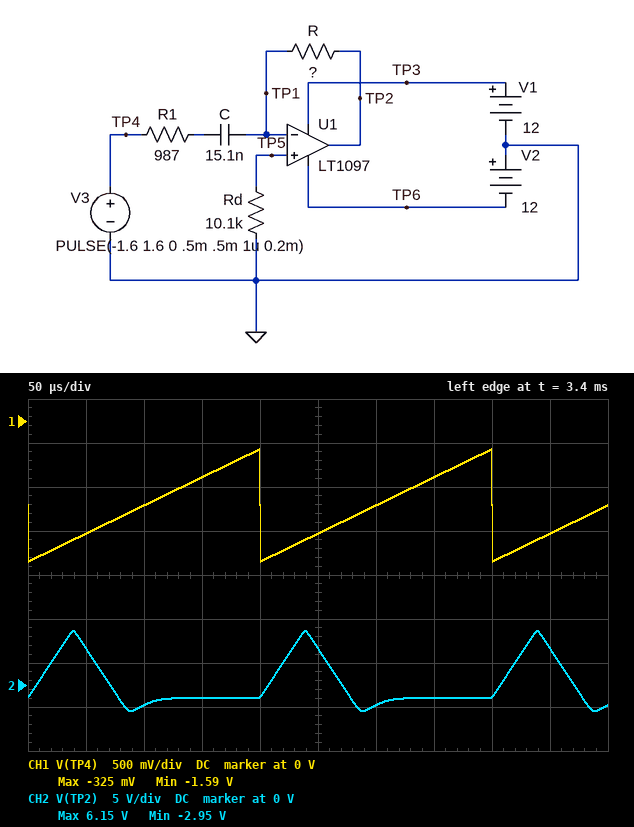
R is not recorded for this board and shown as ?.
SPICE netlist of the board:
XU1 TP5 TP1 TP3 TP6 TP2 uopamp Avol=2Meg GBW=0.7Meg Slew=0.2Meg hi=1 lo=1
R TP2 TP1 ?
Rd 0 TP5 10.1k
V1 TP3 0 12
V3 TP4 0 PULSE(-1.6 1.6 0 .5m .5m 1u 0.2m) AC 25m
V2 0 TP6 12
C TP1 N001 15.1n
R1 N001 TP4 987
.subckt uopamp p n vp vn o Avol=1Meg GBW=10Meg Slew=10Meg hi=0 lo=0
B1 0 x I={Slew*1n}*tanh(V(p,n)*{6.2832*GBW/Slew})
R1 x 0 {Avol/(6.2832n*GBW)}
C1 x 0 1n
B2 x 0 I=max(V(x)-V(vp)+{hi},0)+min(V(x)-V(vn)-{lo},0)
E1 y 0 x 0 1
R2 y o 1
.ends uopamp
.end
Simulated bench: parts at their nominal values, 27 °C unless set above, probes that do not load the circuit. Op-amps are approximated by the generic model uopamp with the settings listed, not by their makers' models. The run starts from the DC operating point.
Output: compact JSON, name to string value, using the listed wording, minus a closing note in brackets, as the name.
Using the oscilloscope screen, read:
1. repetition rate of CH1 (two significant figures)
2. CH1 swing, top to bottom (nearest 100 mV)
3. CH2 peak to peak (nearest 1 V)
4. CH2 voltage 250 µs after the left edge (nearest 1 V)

{"repetition rate of CH1": "5.0 kHz", "CH1 swing, top to bottom": "1.3 V", "CH2 peak to peak": "9 V", "CH2 voltage 250 µs after the left edge": "4 V"}
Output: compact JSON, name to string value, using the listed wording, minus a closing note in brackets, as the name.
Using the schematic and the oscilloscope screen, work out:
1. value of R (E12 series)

{"value of R": "15 kΩ"}
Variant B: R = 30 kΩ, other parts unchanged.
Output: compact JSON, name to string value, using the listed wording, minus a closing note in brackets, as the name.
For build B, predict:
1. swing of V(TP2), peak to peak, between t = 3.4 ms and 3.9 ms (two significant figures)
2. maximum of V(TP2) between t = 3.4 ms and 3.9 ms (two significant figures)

{"swing of V(TP2), peak to peak, between t = 3.4 ms and 3.9 ms": "17 V", "maximum of V(TP2) between t = 3.4 ms and 3.9 ms": "9.0 V"}
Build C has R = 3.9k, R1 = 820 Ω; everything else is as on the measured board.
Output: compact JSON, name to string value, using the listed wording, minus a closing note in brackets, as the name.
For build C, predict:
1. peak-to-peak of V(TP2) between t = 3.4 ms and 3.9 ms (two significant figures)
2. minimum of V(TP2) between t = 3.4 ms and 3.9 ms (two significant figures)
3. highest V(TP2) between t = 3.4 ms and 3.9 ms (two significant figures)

{"peak-to-peak of V(TP2) between t = 3.4 ms and 3.9 ms": "3.2 V", "minimum of V(TP2) between t = 3.4 ms and 3.9 ms": "-380 mV", "highest V(TP2) between t = 3.4 ms and 3.9 ms": "2.8 V"}
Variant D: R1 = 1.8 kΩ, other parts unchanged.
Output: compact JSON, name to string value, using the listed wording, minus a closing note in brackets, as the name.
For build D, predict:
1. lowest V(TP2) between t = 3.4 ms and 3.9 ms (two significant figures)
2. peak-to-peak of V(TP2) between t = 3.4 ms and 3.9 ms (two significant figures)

{"lowest V(TP2) between t = 3.4 ms and 3.9 ms": "-1.4 V", "peak-to-peak of V(TP2) between t = 3.4 ms and 3.9 ms": "6.2 V"}
